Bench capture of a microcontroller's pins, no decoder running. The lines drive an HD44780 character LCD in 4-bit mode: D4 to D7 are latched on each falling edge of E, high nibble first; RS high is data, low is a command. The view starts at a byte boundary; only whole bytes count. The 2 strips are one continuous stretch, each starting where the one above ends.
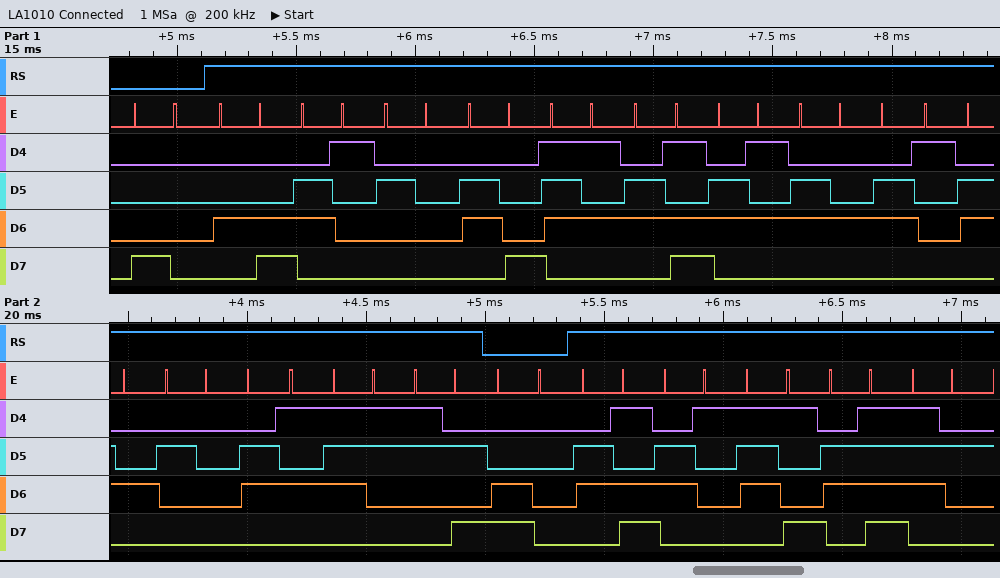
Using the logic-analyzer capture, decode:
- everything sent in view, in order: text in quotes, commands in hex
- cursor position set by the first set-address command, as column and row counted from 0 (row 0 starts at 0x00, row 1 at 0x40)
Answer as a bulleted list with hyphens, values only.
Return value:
- 0x80 "La humedad es:" 0xC0 "mayor"
- column 0, row 0
